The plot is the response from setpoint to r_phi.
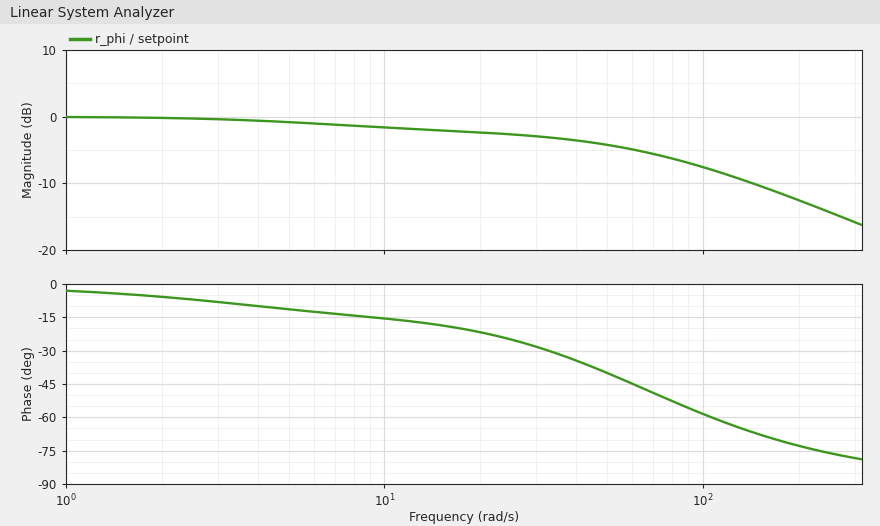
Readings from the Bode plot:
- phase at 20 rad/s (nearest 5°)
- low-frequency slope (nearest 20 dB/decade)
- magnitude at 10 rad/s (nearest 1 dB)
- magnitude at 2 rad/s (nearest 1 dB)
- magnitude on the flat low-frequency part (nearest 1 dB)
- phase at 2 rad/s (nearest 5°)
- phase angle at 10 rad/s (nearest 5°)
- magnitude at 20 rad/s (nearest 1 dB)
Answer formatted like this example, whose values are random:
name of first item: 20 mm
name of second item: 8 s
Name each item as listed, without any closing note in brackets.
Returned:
phase at 20 rad/s: -20°
low-frequency slope: 0 dB/decade
magnitude at 10 rad/s: -2 dB
magnitude at 2 rad/s: 0 dB
magnitude on the flat low-frequency part: 0 dB
phase at 2 rad/s: -5°
phase angle at 10 rad/s: -15°
magnitude at 20 rad/s: -2 dB
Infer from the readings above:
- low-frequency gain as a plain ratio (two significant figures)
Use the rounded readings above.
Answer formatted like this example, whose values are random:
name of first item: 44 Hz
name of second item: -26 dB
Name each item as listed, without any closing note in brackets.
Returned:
low-frequency gain as a plain ratio: 1.0
